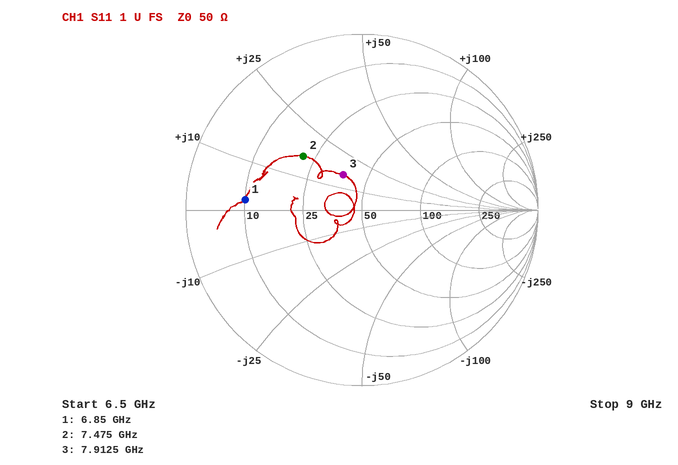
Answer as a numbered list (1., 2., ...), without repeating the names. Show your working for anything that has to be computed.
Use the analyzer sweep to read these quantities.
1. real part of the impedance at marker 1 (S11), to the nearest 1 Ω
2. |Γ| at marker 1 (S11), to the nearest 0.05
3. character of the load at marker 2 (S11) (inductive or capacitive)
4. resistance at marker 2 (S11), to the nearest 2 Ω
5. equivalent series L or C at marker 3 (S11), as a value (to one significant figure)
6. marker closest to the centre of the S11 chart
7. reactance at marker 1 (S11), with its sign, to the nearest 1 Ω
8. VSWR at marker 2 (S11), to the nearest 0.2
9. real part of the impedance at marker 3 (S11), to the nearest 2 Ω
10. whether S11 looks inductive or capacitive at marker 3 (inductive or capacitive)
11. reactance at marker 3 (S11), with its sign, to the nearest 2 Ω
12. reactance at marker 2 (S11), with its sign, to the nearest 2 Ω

1. 10 Ω
2. 0.65
3. inductive
4. 22 Ω
5. L = 16 Ω/(2π × 7.9125 GHz) ≈ 322 pH, so 300 pH to one significant figure
6. marker 3
7. +2 Ω
8. 2.6
9. 38 Ω
10. inductive
11. +16 Ω
12. +16 Ω
